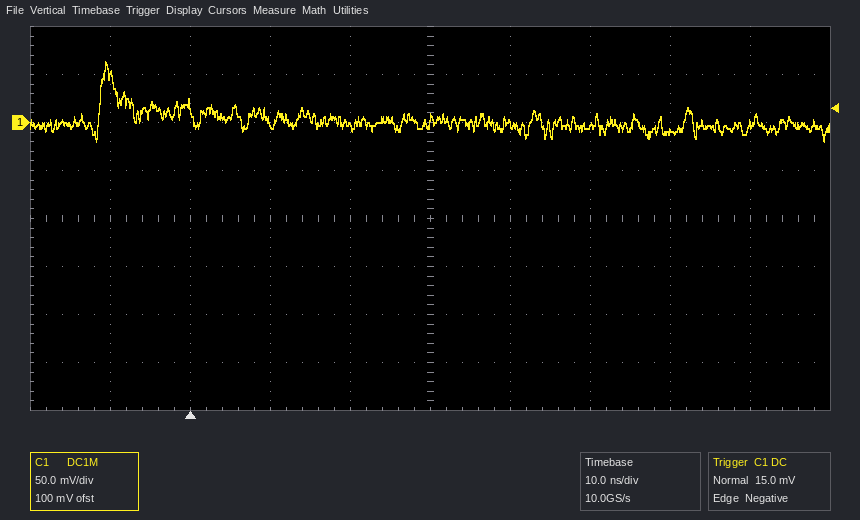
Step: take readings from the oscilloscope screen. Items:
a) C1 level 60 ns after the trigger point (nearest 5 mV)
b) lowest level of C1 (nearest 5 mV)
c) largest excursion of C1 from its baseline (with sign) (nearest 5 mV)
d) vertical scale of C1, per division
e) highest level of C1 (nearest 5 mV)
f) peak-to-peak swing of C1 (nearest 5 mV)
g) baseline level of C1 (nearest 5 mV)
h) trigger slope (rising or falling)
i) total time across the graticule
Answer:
-10 mV
-20 mV
+65 mV
50 mV
65 mV
85 mV
0 mV
falling
100 ns
